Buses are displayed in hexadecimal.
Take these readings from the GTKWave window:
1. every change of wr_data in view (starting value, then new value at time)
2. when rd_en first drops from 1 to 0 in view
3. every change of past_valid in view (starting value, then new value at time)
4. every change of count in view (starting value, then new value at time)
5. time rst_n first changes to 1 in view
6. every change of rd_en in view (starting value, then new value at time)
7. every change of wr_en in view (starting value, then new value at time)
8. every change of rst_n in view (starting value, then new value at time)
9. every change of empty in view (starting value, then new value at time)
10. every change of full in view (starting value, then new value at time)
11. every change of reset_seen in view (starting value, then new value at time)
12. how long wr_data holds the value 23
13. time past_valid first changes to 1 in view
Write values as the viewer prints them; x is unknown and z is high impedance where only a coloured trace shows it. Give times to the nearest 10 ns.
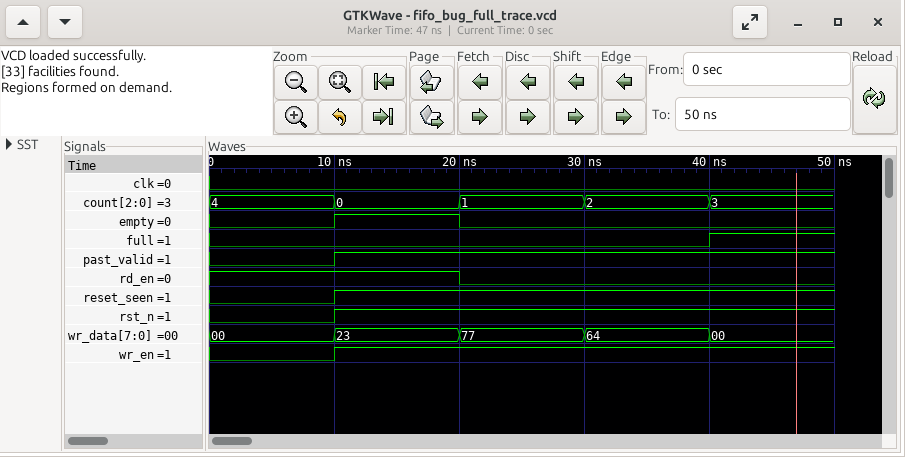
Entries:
00, 23 at 10 ns, 77 at 20 ns, 64 at 30 ns, 00 at 40 ns
20 ns
0, 1 at 10 ns
4, 0 at 10 ns, 1 at 20 ns, 2 at 30 ns, 3 at 40 ns
10 ns
1, 0 at 20 ns
0, 1 at 10 ns
0, 1 at 10 ns
0, 1 at 10 ns, 0 at 20 ns
0, 1 at 40 ns
0, 1 at 10 ns
10 ns
10 ns
